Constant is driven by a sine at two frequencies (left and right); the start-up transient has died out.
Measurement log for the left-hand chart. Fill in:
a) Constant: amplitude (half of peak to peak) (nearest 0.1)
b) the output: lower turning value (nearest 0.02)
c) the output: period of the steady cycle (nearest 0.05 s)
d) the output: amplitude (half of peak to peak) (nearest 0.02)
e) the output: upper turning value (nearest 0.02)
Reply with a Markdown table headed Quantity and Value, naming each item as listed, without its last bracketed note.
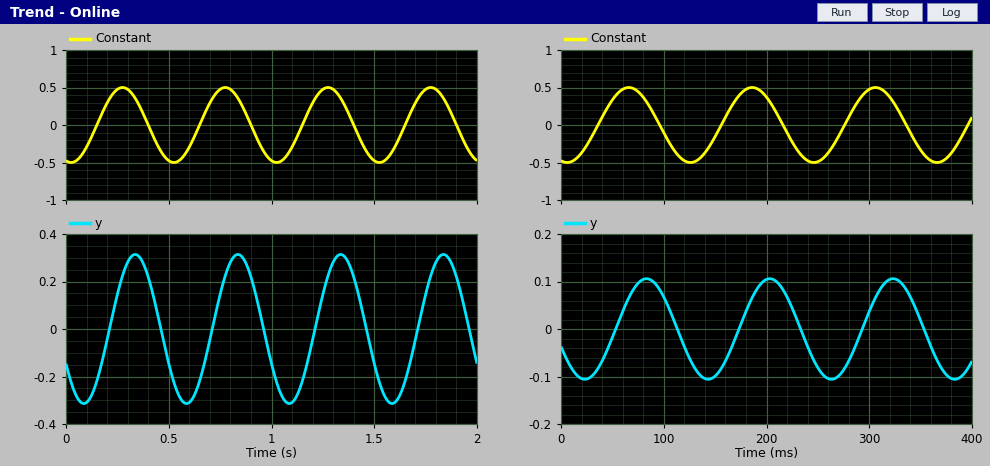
| Quantity | Value |
|---|---|
| Constant: amplitude (half of peak to peak) | 0.5 |
| the output: lower turning value | -0.32 |
| the output: period of the steady cycle | 0.50 s |
| the output: amplitude (half of peak to peak) | 0.32 |
| the output: upper turning value | 0.32 |
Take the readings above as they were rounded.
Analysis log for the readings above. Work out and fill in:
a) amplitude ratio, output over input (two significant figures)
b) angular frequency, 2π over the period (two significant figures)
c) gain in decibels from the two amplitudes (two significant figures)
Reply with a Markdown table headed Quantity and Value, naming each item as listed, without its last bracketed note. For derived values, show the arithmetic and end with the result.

| Quantity | Value |
|---|---|
| amplitude ratio, output over input | 0.32 / 0.5 = 0.64 |
| angular frequency, 2π over the period | 2π / 0.5 = 13 rad/s |
| gain in decibels from the two amplitudes | 20 log10(0.32 / 0.5) = -3.9 dB |
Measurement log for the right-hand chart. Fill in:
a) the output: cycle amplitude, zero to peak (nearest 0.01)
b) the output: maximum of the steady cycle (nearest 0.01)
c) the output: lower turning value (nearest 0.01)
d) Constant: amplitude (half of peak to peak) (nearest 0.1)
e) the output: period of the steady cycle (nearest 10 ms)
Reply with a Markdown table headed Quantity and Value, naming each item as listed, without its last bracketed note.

| Quantity | Value |
|---|---|
| the output: cycle amplitude, zero to peak | 0.11 |
| the output: maximum of the steady cycle | 0.11 |
| the output: lower turning value | -0.11 |
| Constant: amplitude (half of peak to peak) | 0.5 |
| the output: period of the steady cycle | 120 ms |
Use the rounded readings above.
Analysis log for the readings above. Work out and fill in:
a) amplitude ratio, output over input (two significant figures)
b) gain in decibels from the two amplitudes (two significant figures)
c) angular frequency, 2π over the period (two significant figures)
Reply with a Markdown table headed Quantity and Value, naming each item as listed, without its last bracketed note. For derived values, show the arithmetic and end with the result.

| Quantity | Value |
|---|---|
| amplitude ratio, output over input | 0.11 / 0.5 = 0.22 |
| gain in decibels from the two amplitudes | 20 log10(0.11 / 0.5) = -13 dB |
| angular frequency, 2π over the period | 2π / 120 = 0.052 rad/ms |
